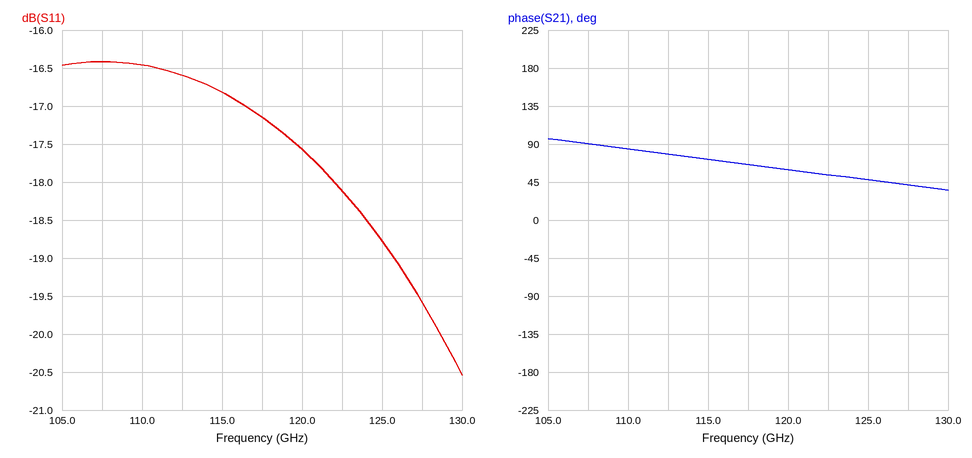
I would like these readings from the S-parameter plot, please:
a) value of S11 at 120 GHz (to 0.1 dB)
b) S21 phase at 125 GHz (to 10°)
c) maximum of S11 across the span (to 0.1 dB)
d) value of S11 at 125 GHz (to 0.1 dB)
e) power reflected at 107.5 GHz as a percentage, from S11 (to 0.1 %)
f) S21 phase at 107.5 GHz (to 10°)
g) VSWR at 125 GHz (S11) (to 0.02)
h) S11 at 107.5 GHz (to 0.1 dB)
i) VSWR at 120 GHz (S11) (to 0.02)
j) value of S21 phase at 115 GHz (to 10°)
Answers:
-17.6 dB
50°
-16.4 dB
-18.8 dB
2.3 %
90°
1.26
-16.4 dB
1.30
70°
